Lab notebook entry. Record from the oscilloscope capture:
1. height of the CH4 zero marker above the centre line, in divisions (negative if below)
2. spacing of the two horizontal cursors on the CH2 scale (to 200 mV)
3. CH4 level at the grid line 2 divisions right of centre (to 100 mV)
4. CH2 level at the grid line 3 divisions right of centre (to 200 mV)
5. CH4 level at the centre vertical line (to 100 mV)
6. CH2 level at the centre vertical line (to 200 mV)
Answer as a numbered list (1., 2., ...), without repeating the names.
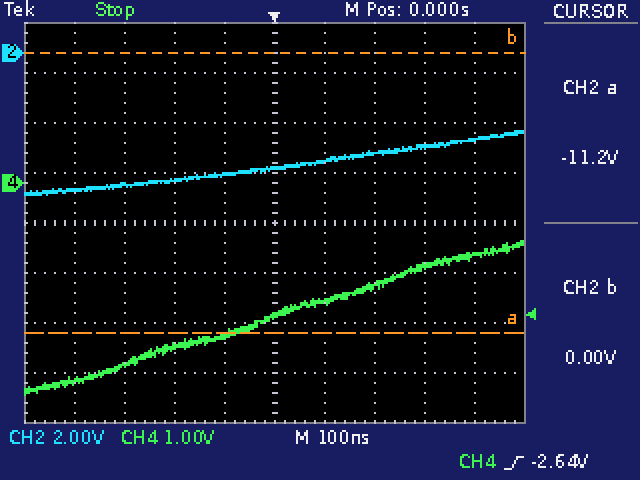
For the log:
1. +0.8 div
2. 11.2 V
3. -2.1 V
4. -3.8 V
5. -2.7 V
6. -4.6 V
